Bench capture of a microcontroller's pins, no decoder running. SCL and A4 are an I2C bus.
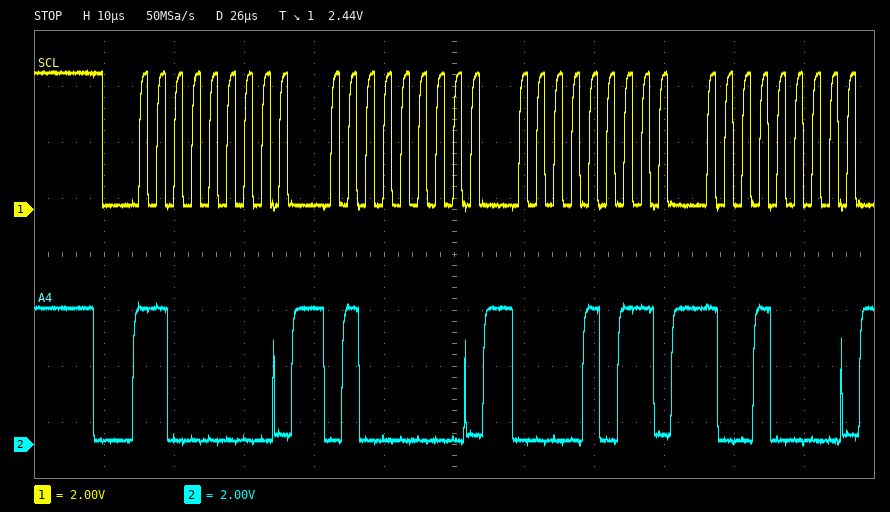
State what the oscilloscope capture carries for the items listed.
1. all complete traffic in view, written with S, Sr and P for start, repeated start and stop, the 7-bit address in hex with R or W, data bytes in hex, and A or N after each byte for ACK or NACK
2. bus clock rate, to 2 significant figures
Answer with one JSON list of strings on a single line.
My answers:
["S 60W A 40 A 0B A 90 A", "400 kHz"]
